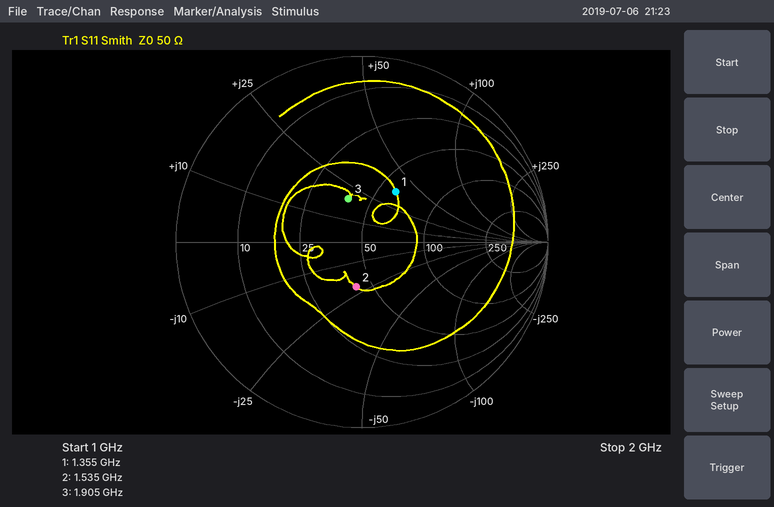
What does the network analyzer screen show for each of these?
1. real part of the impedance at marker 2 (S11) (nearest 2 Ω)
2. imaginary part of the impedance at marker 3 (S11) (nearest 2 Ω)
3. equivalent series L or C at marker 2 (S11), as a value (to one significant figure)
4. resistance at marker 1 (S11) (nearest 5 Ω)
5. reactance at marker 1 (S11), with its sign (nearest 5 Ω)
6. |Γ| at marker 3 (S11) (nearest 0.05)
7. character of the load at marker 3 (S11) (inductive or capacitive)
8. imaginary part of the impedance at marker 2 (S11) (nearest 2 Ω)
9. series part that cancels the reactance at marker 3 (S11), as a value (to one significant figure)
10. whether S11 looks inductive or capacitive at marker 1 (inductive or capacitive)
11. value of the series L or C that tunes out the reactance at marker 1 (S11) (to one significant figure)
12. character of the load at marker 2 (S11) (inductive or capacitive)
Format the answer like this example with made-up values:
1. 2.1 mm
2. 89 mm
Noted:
1. 42 Ω
2. +20 Ω
3. 5 pF
4. 60 Ω
5. +35 Ω
6. 0.25
7. inductive
8. -22 Ω
9. 4 pF
10. inductive
11. 3 pF
12. capacitive
